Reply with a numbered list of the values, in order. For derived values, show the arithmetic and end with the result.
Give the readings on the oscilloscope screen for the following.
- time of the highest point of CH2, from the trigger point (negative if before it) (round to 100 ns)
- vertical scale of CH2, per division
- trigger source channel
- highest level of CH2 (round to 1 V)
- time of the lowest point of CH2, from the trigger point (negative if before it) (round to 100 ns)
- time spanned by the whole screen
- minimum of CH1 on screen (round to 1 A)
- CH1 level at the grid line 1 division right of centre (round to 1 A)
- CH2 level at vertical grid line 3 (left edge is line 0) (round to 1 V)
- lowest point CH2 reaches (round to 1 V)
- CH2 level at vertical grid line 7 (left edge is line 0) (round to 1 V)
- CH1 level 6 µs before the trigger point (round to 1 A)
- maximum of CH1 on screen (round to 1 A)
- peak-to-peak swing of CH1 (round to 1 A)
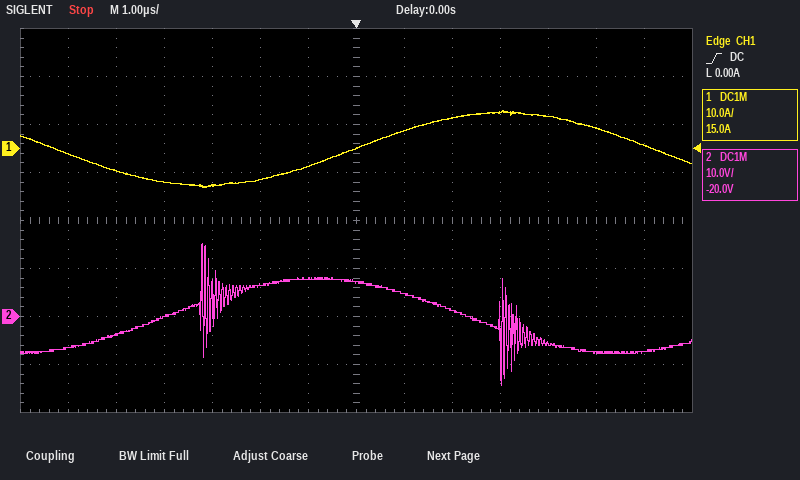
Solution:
1. -3.2 µs
2. 10 V
3. CH1
4. 15 V
5. +3.0 µs
6. 14 µs
7. -8 A
8. 4 A
9. 0 V
10. -14 V
11. 7 V
12. -1 A
13. 8 A
14. 8 A − (-8 A) = 16 A
